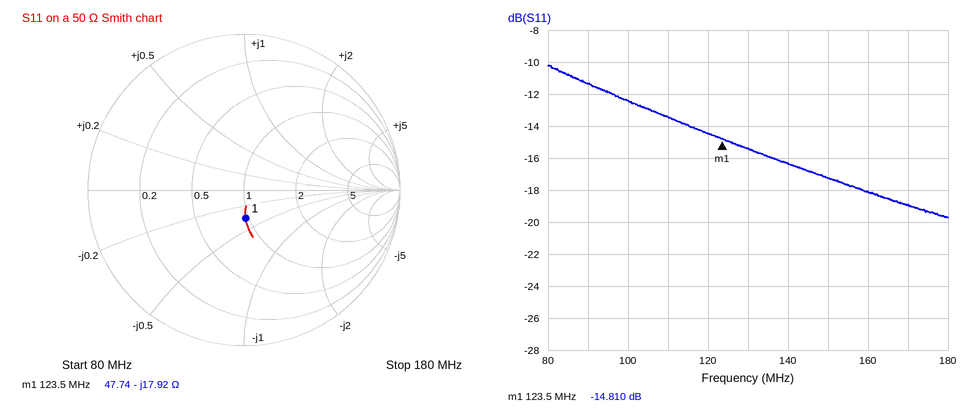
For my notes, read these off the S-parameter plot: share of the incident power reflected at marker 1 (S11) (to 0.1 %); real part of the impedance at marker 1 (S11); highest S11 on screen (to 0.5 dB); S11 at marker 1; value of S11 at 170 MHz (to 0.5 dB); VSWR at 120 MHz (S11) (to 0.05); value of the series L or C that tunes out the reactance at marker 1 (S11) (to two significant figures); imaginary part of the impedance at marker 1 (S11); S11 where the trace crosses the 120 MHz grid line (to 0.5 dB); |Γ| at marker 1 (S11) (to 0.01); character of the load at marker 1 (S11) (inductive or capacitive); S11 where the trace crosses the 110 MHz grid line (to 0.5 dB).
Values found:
3.3 %
47.74 Ω
-10.0 dB
-14.810 dB
-19.0 dB
1.45
23 nH
-17.92 Ω
-14.5 dB
0.18
capacitive
-13.5 dB
